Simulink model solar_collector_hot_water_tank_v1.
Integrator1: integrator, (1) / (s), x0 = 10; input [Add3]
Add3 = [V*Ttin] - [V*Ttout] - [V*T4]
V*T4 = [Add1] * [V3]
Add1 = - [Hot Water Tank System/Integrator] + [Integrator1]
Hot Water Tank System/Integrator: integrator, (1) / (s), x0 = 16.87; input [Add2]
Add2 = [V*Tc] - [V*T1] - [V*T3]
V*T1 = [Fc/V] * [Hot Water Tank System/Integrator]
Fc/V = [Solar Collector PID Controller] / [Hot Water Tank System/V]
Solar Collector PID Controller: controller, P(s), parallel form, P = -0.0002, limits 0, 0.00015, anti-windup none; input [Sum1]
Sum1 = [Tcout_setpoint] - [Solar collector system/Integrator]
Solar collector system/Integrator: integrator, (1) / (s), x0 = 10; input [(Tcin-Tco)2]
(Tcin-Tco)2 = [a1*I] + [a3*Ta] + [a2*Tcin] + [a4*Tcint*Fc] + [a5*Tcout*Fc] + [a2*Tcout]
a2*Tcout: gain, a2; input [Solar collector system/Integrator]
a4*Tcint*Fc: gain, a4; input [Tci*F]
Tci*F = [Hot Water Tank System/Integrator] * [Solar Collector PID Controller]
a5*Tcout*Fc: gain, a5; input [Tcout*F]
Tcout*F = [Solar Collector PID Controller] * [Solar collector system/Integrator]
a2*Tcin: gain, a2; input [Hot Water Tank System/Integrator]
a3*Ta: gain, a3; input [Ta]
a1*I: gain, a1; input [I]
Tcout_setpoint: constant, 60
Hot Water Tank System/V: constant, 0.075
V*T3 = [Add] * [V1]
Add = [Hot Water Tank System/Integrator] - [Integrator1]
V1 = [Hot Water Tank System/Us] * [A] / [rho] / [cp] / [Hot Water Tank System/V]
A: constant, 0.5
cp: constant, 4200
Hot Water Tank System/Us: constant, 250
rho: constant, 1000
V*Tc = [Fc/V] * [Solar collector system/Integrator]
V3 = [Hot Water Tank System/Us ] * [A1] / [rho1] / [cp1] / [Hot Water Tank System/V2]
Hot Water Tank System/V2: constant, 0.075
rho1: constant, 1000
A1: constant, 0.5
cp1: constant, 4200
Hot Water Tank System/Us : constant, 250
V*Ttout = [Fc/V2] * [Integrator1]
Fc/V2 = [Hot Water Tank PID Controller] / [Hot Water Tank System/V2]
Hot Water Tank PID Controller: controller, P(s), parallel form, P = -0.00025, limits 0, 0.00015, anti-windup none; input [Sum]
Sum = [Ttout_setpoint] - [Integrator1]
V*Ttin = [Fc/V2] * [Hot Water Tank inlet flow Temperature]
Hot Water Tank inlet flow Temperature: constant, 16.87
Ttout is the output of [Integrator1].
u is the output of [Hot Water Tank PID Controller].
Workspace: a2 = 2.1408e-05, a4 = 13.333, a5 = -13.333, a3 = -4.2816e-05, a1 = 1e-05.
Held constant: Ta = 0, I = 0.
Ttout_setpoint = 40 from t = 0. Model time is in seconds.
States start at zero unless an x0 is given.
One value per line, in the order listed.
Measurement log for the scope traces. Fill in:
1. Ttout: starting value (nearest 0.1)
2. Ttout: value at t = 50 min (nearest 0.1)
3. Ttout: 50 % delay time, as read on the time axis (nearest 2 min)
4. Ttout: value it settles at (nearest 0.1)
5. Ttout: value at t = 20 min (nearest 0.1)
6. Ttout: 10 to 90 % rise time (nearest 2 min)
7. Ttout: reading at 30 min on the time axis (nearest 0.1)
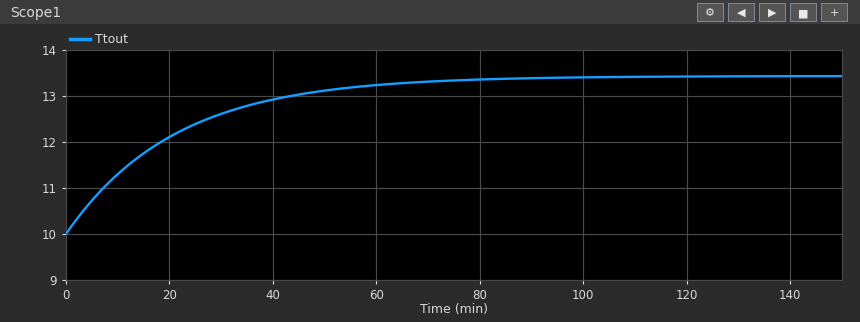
10.0
13.1
14 min
13.4
12.1
46 min
12.6
